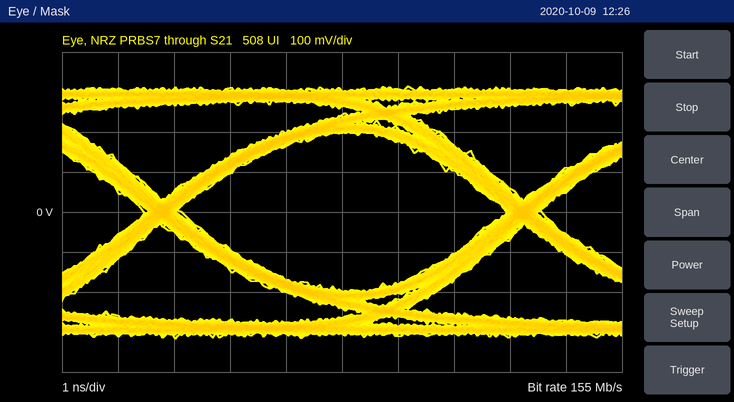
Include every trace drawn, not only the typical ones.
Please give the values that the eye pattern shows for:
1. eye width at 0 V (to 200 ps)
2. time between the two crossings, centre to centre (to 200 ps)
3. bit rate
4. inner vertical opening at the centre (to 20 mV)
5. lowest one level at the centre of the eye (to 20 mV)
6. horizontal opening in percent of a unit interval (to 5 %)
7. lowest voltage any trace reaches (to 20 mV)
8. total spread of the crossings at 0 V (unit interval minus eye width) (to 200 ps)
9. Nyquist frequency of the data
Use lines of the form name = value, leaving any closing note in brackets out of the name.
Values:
eye width at 0 V = 5.8 ns
time between the two crossings, centre to centre = 6.4 ns
bit rate = 155 Mb/s
inner vertical opening at the centre = 400 mV
lowest one level at the centre of the eye = 200 mV
horizontal opening in percent of a unit interval = 90 %
lowest voltage any trace reaches = -320 mV
total spread of the crossings at 0 V (unit interval minus eye width) = 600 ps
Nyquist frequency of the data = 77.5 MHz
